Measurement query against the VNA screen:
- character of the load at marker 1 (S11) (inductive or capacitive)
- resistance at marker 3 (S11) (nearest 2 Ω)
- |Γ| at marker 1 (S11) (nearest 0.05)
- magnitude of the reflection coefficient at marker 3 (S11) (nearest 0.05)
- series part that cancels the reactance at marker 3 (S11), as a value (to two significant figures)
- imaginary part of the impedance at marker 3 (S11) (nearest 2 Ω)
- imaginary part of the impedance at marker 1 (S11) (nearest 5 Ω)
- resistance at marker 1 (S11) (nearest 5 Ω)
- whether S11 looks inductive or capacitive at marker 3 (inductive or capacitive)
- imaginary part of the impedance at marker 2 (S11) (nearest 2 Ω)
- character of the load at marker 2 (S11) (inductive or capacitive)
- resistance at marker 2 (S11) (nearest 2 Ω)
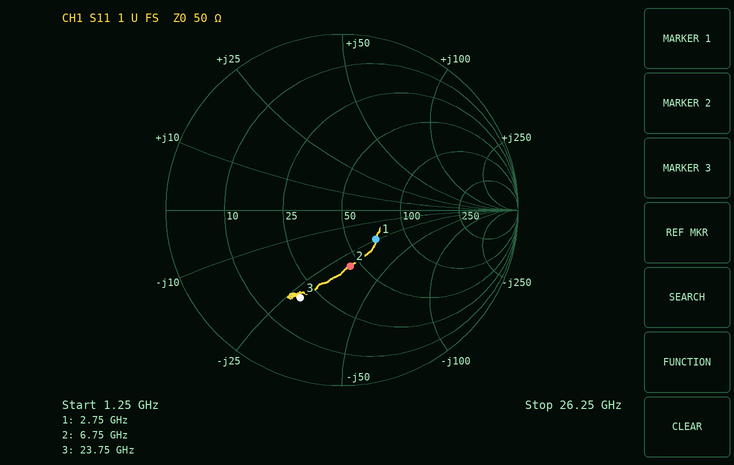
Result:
capacitive
20 Ω
0.25
0.55
190 pH
-28 Ω
-25 Ω
70 Ω
capacitive
-32 Ω
capacitive
44 Ω
